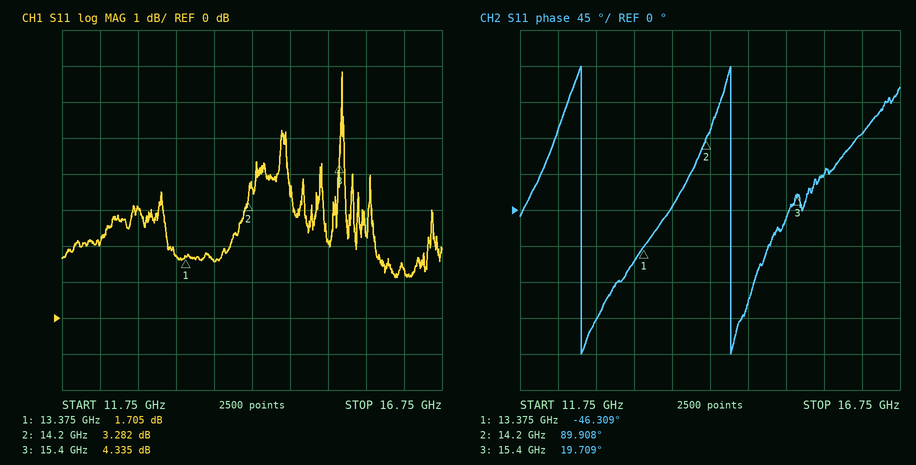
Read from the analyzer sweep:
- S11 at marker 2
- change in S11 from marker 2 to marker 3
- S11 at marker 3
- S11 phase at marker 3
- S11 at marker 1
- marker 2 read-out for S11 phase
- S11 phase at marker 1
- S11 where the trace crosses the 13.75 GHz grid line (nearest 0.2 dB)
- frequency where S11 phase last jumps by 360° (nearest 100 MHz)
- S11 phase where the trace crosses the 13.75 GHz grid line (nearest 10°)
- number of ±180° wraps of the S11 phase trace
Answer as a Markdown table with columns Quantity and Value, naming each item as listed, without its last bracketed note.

| Quantity | Value |
|---|---|
| S11 at marker 2 | 3.282 dB |
| change in S11 from marker 2 to marker 3 | 1.053 dB |
| S11 at marker 3 | 4.335 dB |
| S11 phase at marker 3 | 19.709° |
| S11 at marker 1 | 1.705 dB |
| marker 2 read-out for S11 phase | 89.908° |
| S11 phase at marker 1 | -46.309° |
| S11 where the trace crosses the 13.75 GHz grid line | 1.6 dB |
| frequency where S11 phase last jumps by 360° | 14.5 GHz |
| S11 phase where the trace crosses the 13.75 GHz grid line | 0° |
| number of ±180° wraps of the S11 phase trace | 2 |
